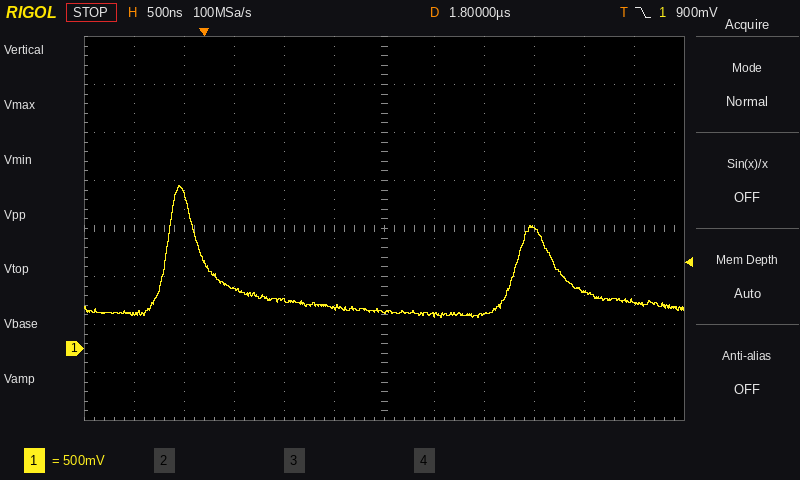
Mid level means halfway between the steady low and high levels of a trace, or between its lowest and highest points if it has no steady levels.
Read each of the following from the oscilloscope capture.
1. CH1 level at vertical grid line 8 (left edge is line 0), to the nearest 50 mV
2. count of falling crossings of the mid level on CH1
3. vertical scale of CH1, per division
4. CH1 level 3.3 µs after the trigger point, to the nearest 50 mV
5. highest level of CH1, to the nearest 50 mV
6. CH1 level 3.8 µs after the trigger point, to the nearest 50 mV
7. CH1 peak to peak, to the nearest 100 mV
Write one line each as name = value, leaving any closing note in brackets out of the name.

CH1 level at vertical grid line 8 (left edge is line 0), to the nearest 50 mV = 350 mV
count of falling crossings of the mid level on CH1 = 2
vertical scale of CH1, per division = 500 mV
CH1 level 3.3 µs after the trigger point, to the nearest 50 mV = 1.25 V
highest level of CH1, to the nearest 50 mV = 1.70 V
CH1 level 3.8 µs after the trigger point, to the nearest 50 mV = 600 mV
CH1 peak to peak, to the nearest 100 mV = 1.40 V
